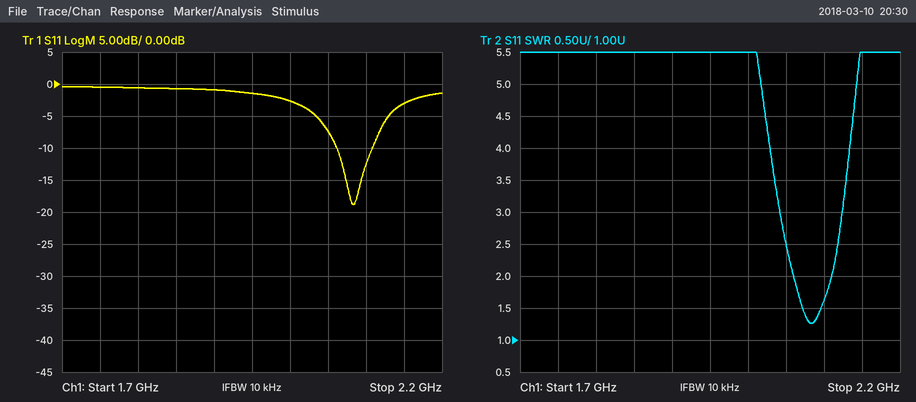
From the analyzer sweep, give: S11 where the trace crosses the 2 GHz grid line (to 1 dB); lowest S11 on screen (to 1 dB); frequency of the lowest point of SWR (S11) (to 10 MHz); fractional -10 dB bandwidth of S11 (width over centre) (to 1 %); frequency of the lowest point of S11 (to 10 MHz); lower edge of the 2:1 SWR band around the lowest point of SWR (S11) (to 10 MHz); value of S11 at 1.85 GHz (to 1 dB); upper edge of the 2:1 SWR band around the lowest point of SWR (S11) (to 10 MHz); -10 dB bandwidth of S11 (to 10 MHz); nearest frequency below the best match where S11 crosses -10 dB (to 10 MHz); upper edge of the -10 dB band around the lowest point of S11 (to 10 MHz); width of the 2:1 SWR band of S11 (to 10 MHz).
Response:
-3 dB
-19 dB
2.08 GHz
2 %
2.08 GHz
2.06 GHz
-1 dB
2.11 GHz
50 MHz
2.06 GHz
2.11 GHz
50 MHz
